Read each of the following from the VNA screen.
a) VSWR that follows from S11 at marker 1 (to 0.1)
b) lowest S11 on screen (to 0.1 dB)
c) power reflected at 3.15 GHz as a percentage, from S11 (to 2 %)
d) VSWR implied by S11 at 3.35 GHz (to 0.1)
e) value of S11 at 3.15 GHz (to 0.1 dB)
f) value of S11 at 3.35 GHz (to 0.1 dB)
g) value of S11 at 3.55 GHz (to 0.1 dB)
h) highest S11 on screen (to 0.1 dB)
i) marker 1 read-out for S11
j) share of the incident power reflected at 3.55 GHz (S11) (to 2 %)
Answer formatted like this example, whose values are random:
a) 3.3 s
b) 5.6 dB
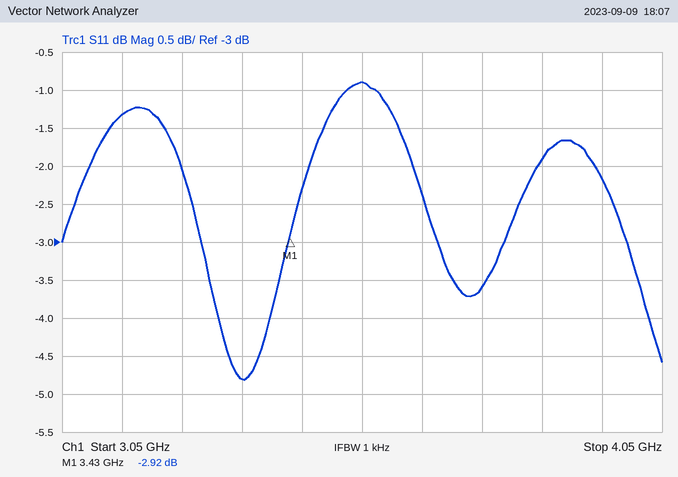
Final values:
a) 6.0
b) -4.8 dB
c) 74 %
d) 3.7
e) -1.3 dB
f) -4.8 dB
g) -0.9 dB
h) -0.9 dB
i) -2.92 dB
j) 82 %
